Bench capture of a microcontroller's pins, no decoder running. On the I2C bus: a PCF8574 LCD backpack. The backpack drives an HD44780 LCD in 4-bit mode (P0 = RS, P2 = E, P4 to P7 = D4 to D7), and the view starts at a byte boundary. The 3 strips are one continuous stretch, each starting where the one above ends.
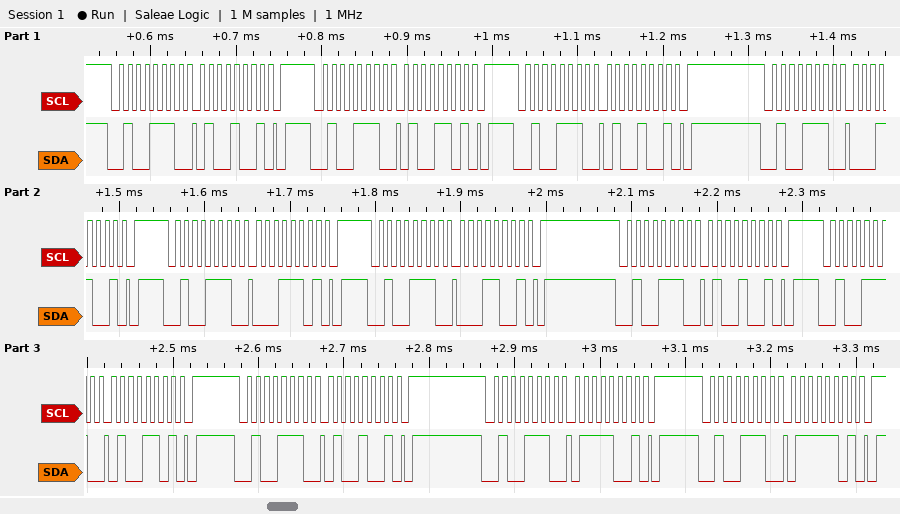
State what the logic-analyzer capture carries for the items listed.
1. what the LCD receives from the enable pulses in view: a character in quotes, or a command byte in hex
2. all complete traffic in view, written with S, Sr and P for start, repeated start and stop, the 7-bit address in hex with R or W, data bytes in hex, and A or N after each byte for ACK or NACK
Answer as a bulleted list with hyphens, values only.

- 'A'
- S 27W A 49 A P S 27W A 4D A P S 27W A 49 A P S 27W A 19 A P S 27W A 1D A P S 27W A 19 A P S 27W A 49 A P S 27W A 4D A P S 27W A 49 A P S 27W A 79 A P S 27W A 7D A P
